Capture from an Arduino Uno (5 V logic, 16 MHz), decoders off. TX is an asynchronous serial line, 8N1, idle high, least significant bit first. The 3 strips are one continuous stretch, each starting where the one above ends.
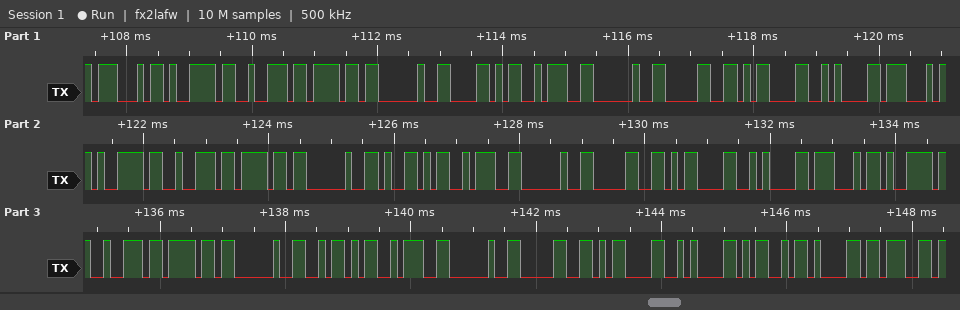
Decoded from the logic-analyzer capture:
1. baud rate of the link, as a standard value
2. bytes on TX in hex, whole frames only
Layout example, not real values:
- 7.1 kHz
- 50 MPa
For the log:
- 9600 baud
- 0x47 0x79 0x72 0x6F 0x20 0x58 0x3A 0x20 0x30 0x0D 0x0A 0x47 0x79 0x72 0x6F 0x20 0x59 0x3A 0x20 0x30 0x0D 0x0A 0x47 0x79 0x72 0x6F 0x20 0x5A 0x3A 0x20 0x30 0x0D 0x0A 0x4D 0x61 0x67
